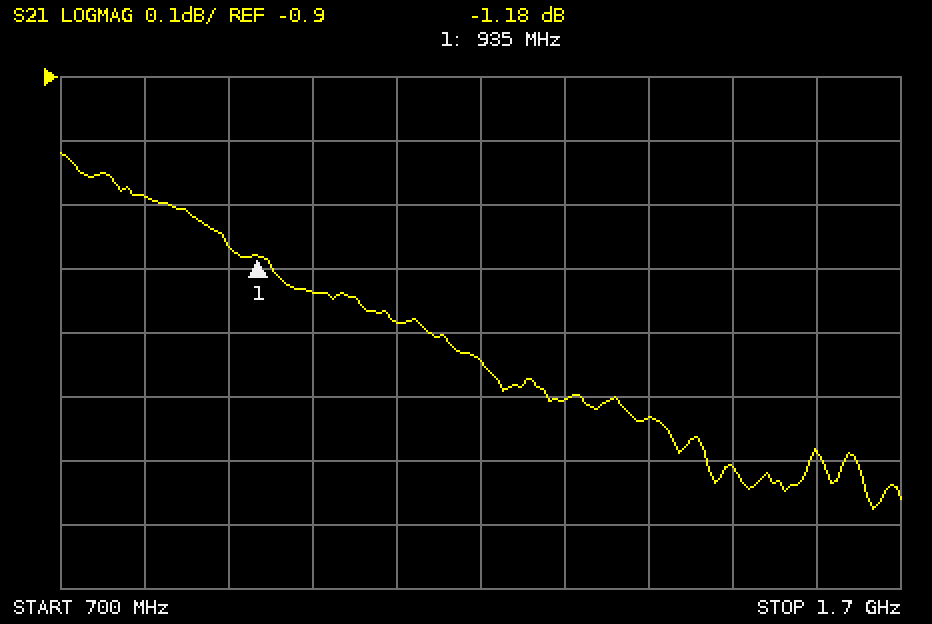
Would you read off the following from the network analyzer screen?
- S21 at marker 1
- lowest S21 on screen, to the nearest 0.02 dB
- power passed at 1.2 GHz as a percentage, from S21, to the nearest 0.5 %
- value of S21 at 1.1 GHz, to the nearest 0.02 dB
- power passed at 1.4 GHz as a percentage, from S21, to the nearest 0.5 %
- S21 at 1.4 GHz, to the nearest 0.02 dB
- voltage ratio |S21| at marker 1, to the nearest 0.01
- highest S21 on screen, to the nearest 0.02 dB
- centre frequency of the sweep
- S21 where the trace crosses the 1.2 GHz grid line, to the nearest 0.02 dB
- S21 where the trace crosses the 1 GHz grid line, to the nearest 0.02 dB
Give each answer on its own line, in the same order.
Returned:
-1.18 dB
-1.58 dB
73.5 %
-1.28 dB
72.0 %
-1.44 dB
0.87
-1.02 dB
1.2 GHz
-1.34 dB
-1.24 dB
